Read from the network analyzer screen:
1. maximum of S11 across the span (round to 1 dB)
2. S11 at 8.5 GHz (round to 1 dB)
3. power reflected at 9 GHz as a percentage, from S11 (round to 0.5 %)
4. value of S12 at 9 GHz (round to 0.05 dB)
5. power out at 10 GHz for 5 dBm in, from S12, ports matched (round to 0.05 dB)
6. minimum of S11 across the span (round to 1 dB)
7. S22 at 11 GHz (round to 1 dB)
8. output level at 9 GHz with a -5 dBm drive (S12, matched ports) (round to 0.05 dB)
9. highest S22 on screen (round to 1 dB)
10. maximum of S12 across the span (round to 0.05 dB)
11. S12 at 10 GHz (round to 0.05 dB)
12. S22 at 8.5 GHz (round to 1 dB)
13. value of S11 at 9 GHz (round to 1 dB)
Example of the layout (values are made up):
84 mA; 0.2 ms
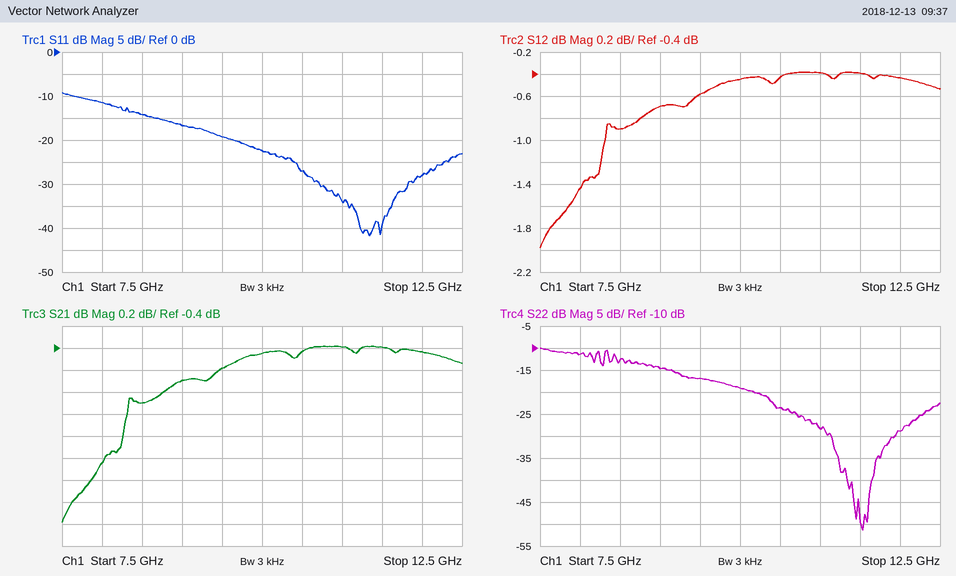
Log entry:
-9 dB; -14 dB; 2.0 %; -0.70 dB; 4.55 dBm; -42 dB; -28 dB; -5.70 dBm; -10 dB; -0.40 dB; -0.45 dB; -13 dB; -17 dB
